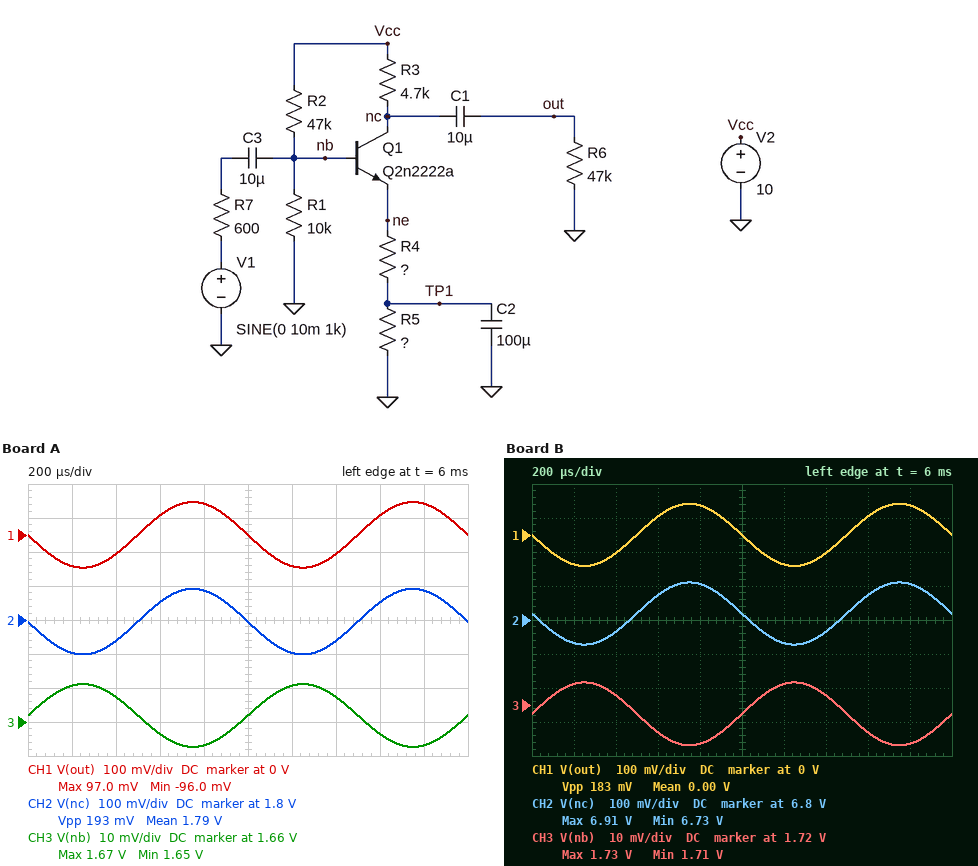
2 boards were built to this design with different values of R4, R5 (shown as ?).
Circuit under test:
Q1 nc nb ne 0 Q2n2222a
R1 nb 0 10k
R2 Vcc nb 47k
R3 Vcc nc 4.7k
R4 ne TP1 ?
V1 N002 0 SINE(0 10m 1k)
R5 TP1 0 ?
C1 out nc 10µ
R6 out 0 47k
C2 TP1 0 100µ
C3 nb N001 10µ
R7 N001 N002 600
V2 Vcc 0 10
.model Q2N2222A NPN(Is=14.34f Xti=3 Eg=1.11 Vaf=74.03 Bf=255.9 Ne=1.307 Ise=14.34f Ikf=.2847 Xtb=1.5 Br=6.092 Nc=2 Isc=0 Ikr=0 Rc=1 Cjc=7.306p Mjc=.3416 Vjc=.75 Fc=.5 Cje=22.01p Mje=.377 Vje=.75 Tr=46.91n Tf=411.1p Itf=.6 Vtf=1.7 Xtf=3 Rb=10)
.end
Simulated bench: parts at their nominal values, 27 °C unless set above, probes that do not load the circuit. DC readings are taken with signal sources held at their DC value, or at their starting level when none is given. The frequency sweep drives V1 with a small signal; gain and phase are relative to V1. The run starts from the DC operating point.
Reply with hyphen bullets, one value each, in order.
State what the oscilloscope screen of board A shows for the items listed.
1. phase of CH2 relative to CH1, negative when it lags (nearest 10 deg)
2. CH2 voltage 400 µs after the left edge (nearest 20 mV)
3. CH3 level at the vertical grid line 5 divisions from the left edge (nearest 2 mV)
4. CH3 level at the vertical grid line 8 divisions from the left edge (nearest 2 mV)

- 0 deg
- 1.74 V
- 1.662 V
- 1.656 V
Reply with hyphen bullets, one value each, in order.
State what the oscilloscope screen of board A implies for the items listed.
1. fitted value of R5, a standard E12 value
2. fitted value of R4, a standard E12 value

- 180 Ω
- 390 Ω
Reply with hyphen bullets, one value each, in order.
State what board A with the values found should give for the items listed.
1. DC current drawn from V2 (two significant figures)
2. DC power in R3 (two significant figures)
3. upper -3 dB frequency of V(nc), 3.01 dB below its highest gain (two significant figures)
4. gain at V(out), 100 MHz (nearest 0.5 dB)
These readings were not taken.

- 1.9 mA
- 14 mW
- 2.1 MHz
- -6.5 dB
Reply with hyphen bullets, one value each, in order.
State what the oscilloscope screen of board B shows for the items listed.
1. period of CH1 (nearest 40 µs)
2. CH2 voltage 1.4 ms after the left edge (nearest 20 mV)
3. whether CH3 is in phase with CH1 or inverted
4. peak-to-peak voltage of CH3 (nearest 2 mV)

- 1.00 ms
- 6.76 V
- inverted
- 18 mV
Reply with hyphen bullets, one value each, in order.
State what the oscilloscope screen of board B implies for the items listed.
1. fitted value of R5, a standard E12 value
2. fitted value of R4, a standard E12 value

- 1.2 kΩ
- 390 Ω
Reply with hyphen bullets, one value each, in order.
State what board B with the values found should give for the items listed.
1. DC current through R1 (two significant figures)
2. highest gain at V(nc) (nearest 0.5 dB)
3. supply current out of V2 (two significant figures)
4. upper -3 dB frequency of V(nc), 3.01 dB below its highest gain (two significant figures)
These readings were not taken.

- 170 µA
- 19.0 dB
- 850 µA
- 4.0 MHz
